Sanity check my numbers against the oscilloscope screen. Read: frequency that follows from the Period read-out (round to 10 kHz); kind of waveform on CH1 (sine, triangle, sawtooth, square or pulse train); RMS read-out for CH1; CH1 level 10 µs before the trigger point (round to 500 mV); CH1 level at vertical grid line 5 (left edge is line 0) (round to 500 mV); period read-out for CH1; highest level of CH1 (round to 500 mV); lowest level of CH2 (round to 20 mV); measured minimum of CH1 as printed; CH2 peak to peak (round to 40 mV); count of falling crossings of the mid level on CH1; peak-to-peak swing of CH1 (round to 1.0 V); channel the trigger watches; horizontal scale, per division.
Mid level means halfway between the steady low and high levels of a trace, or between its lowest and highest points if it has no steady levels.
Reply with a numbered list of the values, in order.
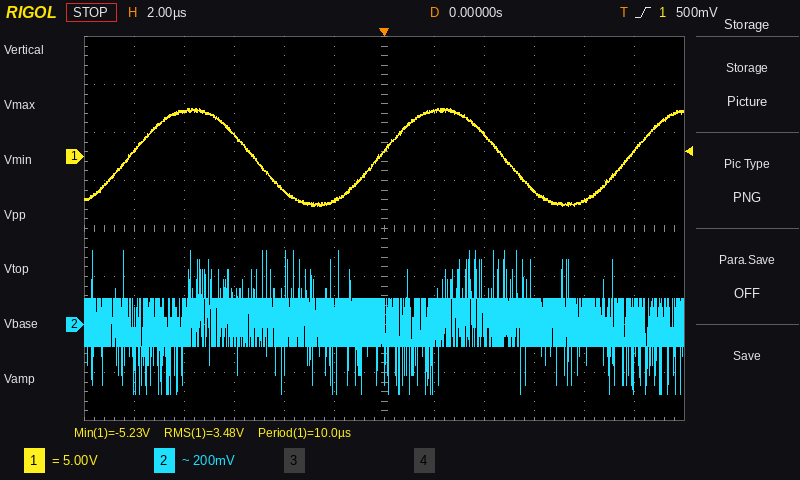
1. 100 kHz
2. sine
3. 3.48 V
4. 500 mV
5. -4.5 V
6. 10.0 µs
7. 5.0 V
8. -300 mV
9. -5.23 V
10. 600 mV
11. 2
12. 10.0 V
13. CH1
14. 2 µs
